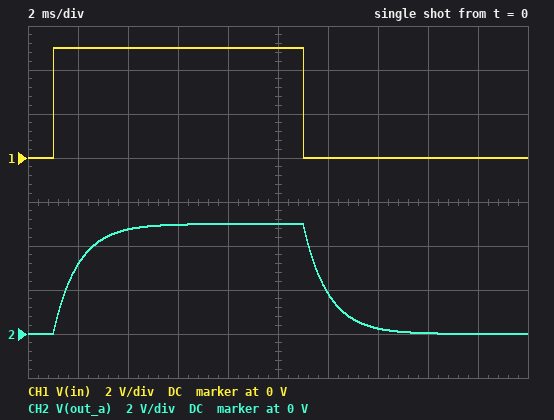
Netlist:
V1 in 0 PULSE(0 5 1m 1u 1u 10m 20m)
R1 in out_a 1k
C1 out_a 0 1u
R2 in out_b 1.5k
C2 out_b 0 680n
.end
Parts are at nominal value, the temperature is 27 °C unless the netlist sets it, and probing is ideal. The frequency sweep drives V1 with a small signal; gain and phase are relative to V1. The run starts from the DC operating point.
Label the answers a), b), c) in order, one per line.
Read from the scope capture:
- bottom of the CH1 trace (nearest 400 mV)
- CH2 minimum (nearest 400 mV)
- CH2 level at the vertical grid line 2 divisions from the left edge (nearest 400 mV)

a) 0 V
b) 0 V
c) 4.8 V
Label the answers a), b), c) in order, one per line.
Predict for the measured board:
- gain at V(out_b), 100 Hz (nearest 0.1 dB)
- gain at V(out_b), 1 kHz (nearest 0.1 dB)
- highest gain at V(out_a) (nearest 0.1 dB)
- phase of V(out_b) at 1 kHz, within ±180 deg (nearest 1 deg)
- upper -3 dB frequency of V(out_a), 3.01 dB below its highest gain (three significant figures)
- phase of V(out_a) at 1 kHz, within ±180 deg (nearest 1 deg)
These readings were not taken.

a) -1.5 dB
b) -16.2 dB
c) 0 dB
d) -81 deg
e) 159 Hz
f) -81 deg
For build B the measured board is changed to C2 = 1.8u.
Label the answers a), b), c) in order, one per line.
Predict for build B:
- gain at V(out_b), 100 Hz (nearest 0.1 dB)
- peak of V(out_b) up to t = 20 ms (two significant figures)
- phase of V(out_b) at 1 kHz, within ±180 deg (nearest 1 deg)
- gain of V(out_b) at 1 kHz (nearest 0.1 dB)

a) -5.9 dB
b) 4.9 V
c) -87 deg
d) -24.6 dB
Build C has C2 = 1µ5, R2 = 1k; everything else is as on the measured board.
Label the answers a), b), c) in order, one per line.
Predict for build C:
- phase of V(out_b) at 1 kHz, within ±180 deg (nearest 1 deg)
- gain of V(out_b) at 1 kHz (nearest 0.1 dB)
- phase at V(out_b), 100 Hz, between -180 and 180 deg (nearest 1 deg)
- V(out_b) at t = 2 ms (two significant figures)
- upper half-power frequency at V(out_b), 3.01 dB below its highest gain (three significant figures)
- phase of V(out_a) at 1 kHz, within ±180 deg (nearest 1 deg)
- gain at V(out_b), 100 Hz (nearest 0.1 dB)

a) -84 deg
b) -19.5 dB
c) -43 deg
d) 2.4 V
e) 106 Hz
f) -81 deg
g) -2.8 dB
